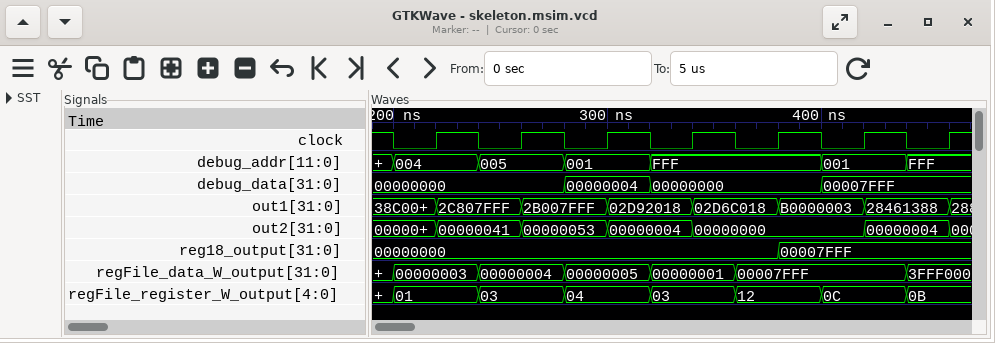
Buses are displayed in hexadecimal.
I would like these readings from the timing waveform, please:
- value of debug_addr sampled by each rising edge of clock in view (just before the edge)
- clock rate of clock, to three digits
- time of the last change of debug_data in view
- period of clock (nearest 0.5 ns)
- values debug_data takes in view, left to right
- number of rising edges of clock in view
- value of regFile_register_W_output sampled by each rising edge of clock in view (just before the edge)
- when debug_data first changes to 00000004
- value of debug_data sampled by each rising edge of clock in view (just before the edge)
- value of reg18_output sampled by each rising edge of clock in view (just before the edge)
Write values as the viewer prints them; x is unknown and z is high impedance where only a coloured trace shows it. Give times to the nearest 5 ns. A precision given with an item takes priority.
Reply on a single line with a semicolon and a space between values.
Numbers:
004, 005, 001, FFF, FFF, 001, FFF; 25.0 MHz; 400 ns; 40 ns; 00000000, 00000004, 00000000, 00007FFF; 7; 01, 03, 04, 03, 12, 0C, 0B; 280 ns; 00000000, 00000000, 00000004, 00000000, 00000000, 00007FFF, 00007FFF; 00000000, 00000000, 00000000, 00000000, 00000000, 00007FFF, 00007FFF
